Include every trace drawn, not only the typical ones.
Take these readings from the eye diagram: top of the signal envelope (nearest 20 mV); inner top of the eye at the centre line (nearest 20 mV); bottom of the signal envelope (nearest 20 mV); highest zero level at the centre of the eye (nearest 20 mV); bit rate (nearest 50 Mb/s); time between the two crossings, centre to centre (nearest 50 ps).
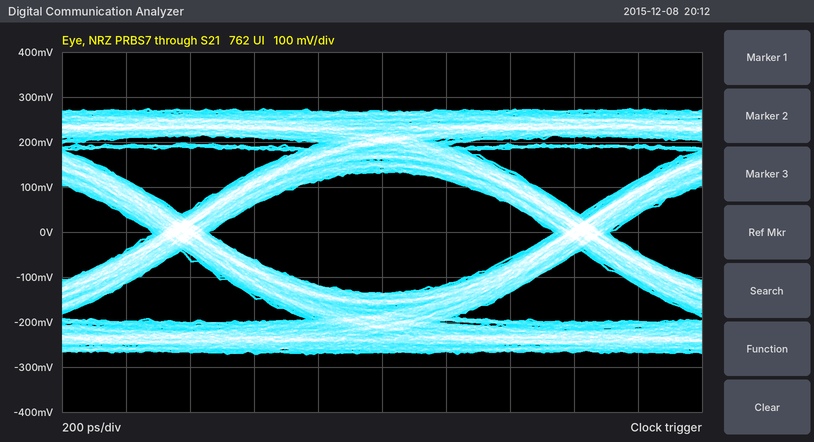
280 mV
140 mV
-280 mV
-140 mV
800 Mb/s
1.25 ns
